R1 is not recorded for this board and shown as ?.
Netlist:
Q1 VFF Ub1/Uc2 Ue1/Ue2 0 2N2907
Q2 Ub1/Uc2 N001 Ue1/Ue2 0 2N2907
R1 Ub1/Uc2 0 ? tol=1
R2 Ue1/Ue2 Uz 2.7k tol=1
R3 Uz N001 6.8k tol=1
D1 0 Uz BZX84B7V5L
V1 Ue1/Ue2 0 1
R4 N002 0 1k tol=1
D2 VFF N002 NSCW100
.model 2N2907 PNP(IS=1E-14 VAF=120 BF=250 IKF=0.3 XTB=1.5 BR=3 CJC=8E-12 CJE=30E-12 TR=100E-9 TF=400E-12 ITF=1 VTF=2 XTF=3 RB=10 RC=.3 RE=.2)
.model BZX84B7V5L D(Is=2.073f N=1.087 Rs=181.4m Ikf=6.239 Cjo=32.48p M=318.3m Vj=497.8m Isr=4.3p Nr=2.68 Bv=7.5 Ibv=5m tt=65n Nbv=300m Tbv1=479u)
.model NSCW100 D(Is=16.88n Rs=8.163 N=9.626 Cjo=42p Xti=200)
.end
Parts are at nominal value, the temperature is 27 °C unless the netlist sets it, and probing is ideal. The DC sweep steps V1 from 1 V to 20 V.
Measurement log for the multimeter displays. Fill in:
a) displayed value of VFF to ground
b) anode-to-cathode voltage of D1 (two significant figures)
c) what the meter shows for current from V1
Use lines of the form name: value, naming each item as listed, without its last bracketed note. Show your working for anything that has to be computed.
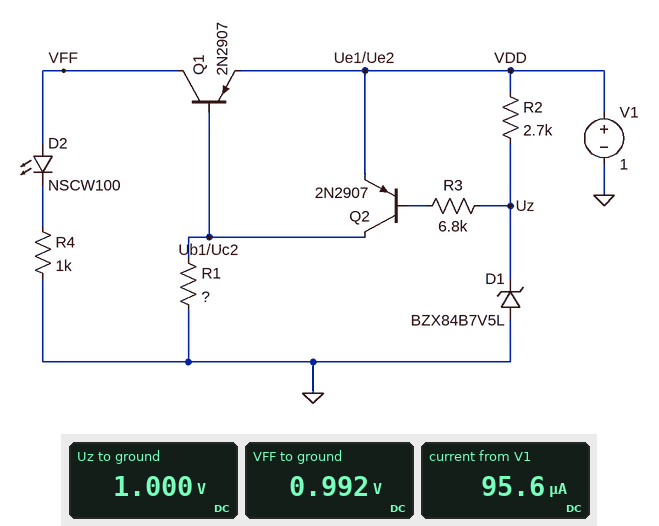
displayed value of VFF to ground: 0.992 V
anode-to-cathode voltage of D1: 0 V - 1 V = -1.0 V
what the meter shows for current from V1: 95.6 µA
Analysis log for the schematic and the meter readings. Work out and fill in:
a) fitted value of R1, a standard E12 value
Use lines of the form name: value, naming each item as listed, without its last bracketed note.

fitted value of R1, a standard E12 value: 3.9 kΩ
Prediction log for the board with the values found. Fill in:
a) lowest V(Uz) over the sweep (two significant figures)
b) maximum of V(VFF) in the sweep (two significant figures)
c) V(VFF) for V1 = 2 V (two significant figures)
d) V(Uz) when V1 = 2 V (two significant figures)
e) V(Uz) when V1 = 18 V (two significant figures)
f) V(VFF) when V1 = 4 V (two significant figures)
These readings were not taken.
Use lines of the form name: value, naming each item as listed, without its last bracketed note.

lowest V(Uz) over the sweep: 1.0 V
maximum of V(VFF) in the sweep: 8.1 V
V(VFF) for V1 = 2 V: 2.0 V
V(Uz) when V1 = 2 V: 2.0 V
V(Uz) when V1 = 18 V: 7.5 V
V(VFF) when V1 = 4 V: 4.0 V
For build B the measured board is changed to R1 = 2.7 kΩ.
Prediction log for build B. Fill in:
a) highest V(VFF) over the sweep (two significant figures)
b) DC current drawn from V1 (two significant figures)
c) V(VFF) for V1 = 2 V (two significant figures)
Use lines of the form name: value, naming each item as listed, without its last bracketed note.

highest V(VFF) over the sweep: 8.2 V
DC current drawn from V1: 130 µA
V(VFF) for V1 = 2 V: 2.0 V
